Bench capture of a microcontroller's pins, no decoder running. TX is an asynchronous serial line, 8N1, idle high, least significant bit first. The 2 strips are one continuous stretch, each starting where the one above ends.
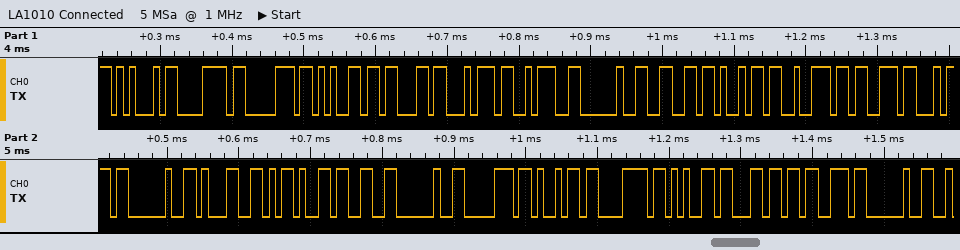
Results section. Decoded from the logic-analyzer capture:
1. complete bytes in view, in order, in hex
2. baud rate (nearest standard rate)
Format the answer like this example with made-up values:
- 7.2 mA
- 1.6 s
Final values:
- 45 78 70 65 63 74 3A 20 66 69 72 73 74 20 31 2D 33 20 70 69 78 65 6C 73 20
- 115200 baud
